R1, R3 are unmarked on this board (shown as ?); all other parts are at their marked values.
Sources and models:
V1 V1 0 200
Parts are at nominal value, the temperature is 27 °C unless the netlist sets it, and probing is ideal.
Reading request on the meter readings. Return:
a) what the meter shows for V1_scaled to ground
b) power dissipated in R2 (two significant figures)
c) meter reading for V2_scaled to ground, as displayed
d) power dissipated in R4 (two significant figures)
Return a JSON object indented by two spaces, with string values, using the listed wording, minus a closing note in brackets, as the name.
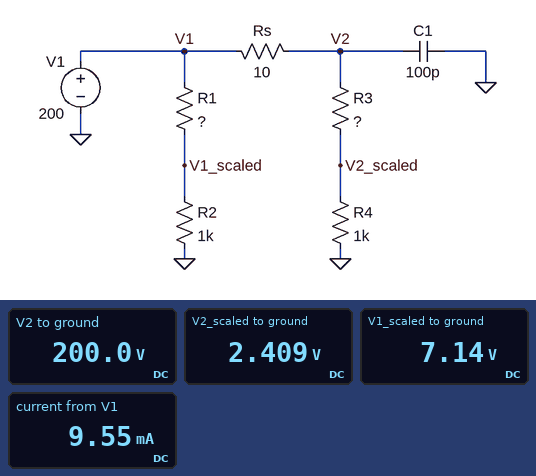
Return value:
{
  "what the meter shows for V1_scaled to ground": "7.14 V",
  "power dissipated in R2": "51 mW",
  "meter reading for V2_scaled to ground, as displayed": "2.409 V",
  "power dissipated in R4": "5.8 mW"
}
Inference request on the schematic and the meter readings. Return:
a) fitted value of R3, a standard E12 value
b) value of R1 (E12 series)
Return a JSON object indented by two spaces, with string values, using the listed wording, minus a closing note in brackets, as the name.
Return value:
{
  "fitted value of R3, a standard E12 value": "82 kΩ",
  "value of R1": "27 kΩ"
}
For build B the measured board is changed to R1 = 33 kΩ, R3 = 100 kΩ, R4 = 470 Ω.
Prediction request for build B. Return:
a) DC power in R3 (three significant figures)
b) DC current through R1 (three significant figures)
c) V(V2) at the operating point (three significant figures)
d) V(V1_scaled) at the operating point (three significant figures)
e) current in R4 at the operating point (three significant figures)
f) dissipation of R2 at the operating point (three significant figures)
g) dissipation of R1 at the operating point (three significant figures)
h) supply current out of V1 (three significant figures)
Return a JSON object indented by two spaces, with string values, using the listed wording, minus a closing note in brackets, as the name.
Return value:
{
  "DC power in R3": "396 mW",
  "DC current through R1": "5.88 mA",
  "V(V2) at the operating point": "200 V",
  "V(V1_scaled) at the operating point": "5.88 V",
  "current in R4 at the operating point": "1.99 mA",
  "dissipation of R2 at the operating point": "34.6 mW",
  "dissipation of R1 at the operating point": "1.14 W",
  "supply current out of V1": "7.87 mA"
}
